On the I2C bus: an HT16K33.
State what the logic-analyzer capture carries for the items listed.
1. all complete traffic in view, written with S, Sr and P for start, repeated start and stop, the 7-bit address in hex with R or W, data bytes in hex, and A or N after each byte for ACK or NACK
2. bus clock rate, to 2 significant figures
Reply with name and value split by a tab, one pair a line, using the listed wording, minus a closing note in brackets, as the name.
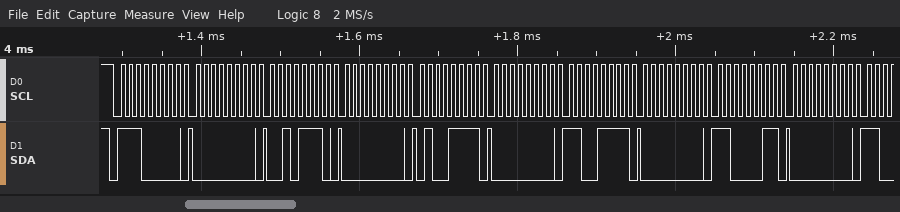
all complete traffic in view, written with S, Sr and P for start, repeated start and stop, the 7-bit address in hex with R or W, data bytes in hex, and A or N after each byte for ACK or NACK	S 70W A 00 A 2E A 00 A 4F A 00 A CF A 00 A C3 A 00 A
bus clock rate, to 2 significant figures	100 kHz
